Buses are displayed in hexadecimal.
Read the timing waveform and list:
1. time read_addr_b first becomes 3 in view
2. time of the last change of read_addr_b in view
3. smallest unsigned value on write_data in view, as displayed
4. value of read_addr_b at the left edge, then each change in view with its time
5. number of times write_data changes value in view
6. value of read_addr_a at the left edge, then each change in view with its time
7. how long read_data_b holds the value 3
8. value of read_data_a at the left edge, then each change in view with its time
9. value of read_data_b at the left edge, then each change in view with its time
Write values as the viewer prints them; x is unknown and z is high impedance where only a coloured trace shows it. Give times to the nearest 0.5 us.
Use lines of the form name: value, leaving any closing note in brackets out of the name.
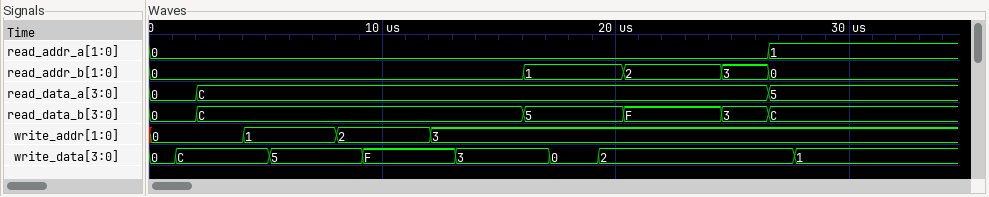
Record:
time read_addr_b first becomes 3 in view: 24.5 us
time of the last change of read_addr_b in view: 26.5 us
smallest unsigned value on write_data in view, as displayed: 0
value of read_addr_b at the left edge, then each change in view with its time: 0, 1 at 16 us, 2 at 20.5 us, 3 at 24.5 us, 0 at 26.5 us
number of times write_data changes value in view: 7
value of read_addr_a at the left edge, then each change in view with its time: 0, 1 at 26.5 us
how long read_data_b holds the value 3: 2 us
value of read_data_a at the left edge, then each change in view with its time: 0, C at 2 us, 5 at 26.5 us
value of read_data_b at the left edge, then each change in view with its time: 0, C at 2 us, 5 at 16 us, F at 20.5 us, 3 at 24.5 us, C at 26.5 us
